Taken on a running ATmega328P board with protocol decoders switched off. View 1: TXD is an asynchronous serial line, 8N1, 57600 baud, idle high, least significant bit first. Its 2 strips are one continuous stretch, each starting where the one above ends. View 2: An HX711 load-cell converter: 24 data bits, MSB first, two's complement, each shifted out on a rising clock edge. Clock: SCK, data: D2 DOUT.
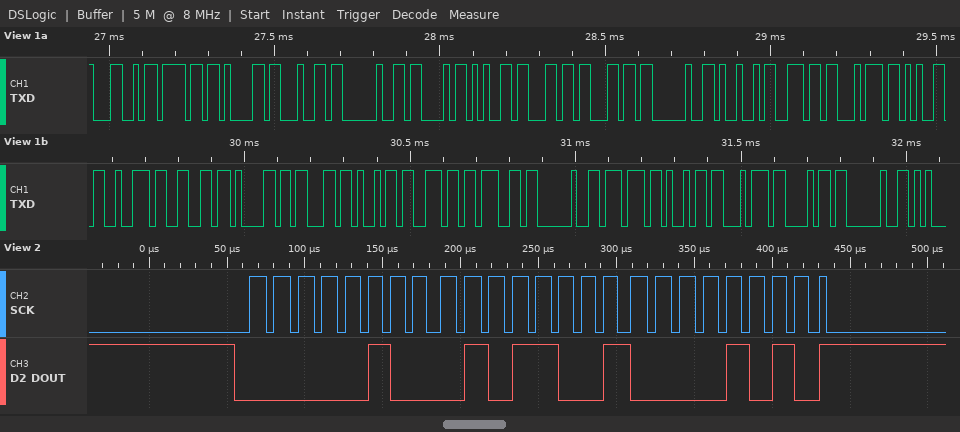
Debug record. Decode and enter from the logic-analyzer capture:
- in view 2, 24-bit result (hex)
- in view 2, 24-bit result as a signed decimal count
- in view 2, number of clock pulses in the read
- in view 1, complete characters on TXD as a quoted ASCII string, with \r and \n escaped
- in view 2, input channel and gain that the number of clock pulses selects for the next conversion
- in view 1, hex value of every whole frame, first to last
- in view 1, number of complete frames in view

0x04590A
284938
25
"Load Cell Interfacing with "
channel A, gain 128
0x4C 0x6F 0x61 0x64 0x20 0x43 0x65 0x6C 0x6C 0x20 0x49 0x6E 0x74 0x65 0x72 0x66 0x61 0x63 0x69 0x6E 0x67 0x20 0x77 0x69 0x74 0x68 0x20
27
